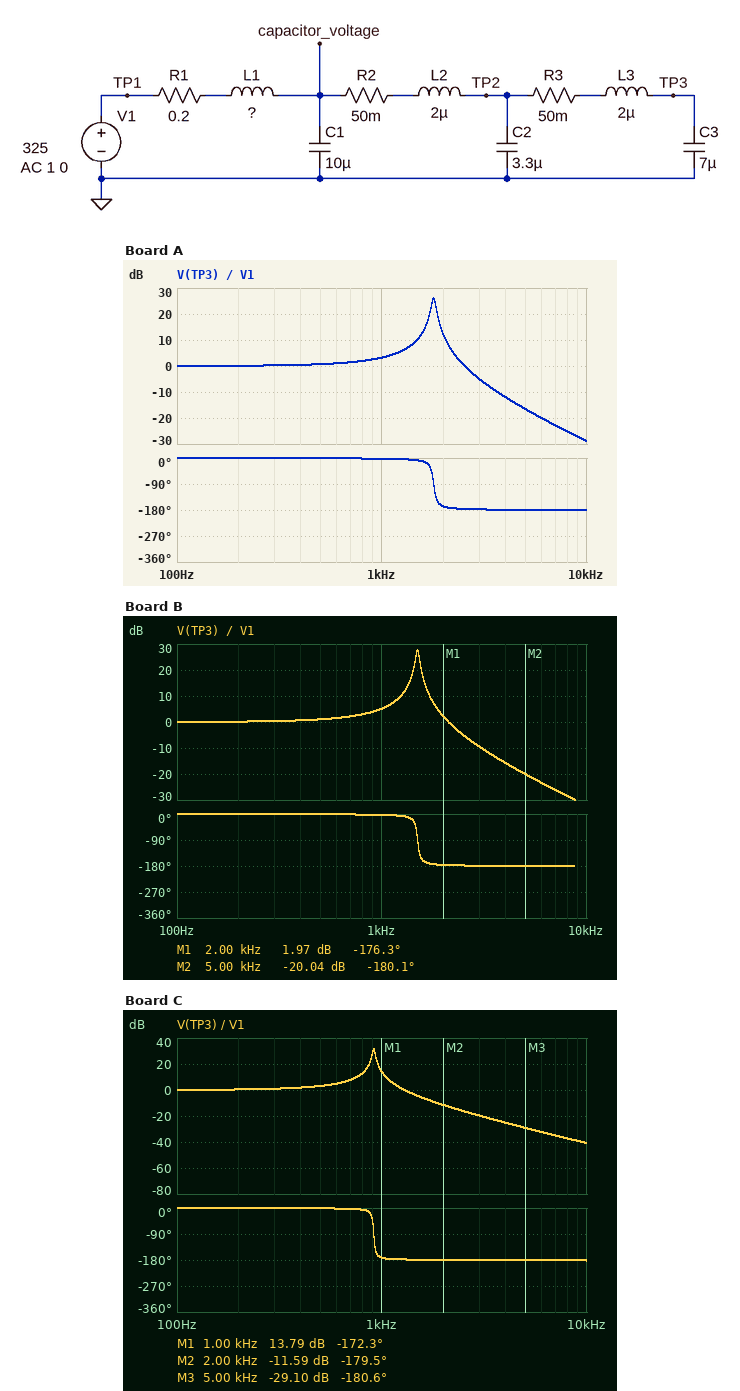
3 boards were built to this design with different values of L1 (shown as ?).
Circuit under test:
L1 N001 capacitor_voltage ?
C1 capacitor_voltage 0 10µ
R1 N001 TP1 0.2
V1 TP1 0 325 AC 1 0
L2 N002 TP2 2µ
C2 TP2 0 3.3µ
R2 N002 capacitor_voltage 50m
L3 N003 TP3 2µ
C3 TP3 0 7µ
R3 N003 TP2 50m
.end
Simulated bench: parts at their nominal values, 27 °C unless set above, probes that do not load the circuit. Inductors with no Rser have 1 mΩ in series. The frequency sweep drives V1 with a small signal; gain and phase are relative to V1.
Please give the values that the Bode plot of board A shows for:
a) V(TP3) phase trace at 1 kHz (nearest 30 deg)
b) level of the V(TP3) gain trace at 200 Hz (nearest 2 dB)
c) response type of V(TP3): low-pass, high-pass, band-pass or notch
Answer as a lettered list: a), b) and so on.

a) 0 deg
b) 0 dB
c) low-pass
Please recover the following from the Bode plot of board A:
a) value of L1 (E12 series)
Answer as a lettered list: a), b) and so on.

a) 390 µH
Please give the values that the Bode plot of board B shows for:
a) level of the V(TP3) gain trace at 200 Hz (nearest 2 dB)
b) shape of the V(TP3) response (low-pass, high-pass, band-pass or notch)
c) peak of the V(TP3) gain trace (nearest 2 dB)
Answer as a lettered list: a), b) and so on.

a) 0 dB
b) low-pass
c) 28 dB
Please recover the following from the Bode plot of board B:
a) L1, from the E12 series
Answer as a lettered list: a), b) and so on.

a) 560 µH
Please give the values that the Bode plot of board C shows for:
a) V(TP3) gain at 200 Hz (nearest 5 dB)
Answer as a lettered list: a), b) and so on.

a) 0 dB
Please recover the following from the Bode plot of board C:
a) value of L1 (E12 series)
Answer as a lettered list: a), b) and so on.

a) 1.5 mH
